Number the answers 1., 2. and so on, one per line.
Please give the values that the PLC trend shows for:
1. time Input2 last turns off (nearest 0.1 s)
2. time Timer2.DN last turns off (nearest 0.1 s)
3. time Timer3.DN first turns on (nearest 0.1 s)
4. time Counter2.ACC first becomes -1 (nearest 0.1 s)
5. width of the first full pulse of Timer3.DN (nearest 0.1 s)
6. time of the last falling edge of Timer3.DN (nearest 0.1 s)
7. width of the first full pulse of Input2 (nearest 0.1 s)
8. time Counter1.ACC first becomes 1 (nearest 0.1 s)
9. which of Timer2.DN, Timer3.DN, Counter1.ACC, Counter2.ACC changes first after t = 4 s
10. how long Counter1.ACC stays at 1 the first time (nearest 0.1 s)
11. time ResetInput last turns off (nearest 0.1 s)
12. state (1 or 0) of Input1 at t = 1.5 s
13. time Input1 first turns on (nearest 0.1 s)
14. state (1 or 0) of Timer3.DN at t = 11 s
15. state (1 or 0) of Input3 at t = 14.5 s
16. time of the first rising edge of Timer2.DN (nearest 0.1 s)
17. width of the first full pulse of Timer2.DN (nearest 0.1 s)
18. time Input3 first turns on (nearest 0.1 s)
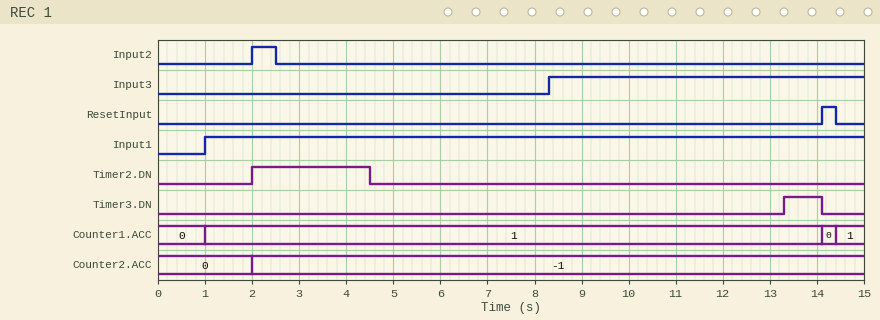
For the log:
1. 2.5 s
2. 4.5 s
3. 13.3 s
4. 2.0 s
5. 0.8 s
6. 14.1 s
7. 0.5 s
8. 1.0 s
9. Timer2.DN
10. 13.1 s
11. 14.4 s
12. 1
13. 1.0 s
14. 0
15. 1
16. 2.0 s
17. 2.5 s
18. 8.3 s
